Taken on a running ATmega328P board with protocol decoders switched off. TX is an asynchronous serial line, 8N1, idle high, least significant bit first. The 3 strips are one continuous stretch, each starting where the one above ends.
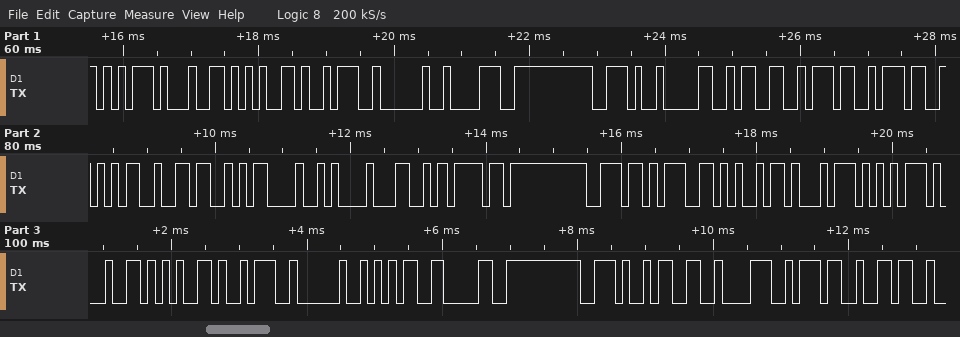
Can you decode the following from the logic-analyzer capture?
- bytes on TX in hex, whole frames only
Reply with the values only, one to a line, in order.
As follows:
0x75 0x64 0x65 0x3A 0x20 0x38 0x2E 0x30 0x33 0x37 0x37 0x35 0x36 0x0D 0x0A 0x4C 0x6F 0x6E 0x67 0x69 0x74 0x75 0x64 0x65 0x3A 0x20 0x35 0x30 0x2E 0x33 0x38 0x37 0x36
